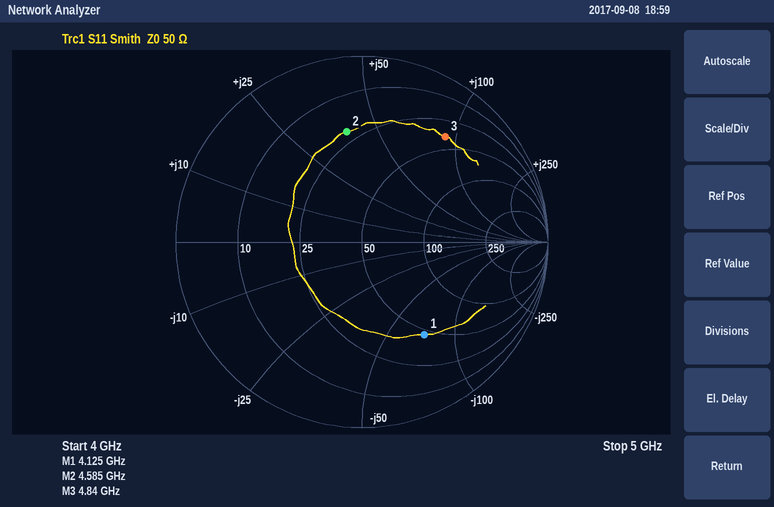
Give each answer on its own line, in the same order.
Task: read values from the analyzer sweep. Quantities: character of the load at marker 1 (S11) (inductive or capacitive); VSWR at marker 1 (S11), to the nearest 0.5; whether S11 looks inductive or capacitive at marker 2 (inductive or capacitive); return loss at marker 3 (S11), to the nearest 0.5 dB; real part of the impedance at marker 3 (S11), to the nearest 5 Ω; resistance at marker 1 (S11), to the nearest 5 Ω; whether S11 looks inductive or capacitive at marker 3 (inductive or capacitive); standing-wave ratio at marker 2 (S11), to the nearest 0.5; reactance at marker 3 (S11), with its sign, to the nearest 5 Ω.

capacitive
4.0
inductive
3.0 dB
40 Ω
45 Ω
inductive
4.0
+90 Ω
